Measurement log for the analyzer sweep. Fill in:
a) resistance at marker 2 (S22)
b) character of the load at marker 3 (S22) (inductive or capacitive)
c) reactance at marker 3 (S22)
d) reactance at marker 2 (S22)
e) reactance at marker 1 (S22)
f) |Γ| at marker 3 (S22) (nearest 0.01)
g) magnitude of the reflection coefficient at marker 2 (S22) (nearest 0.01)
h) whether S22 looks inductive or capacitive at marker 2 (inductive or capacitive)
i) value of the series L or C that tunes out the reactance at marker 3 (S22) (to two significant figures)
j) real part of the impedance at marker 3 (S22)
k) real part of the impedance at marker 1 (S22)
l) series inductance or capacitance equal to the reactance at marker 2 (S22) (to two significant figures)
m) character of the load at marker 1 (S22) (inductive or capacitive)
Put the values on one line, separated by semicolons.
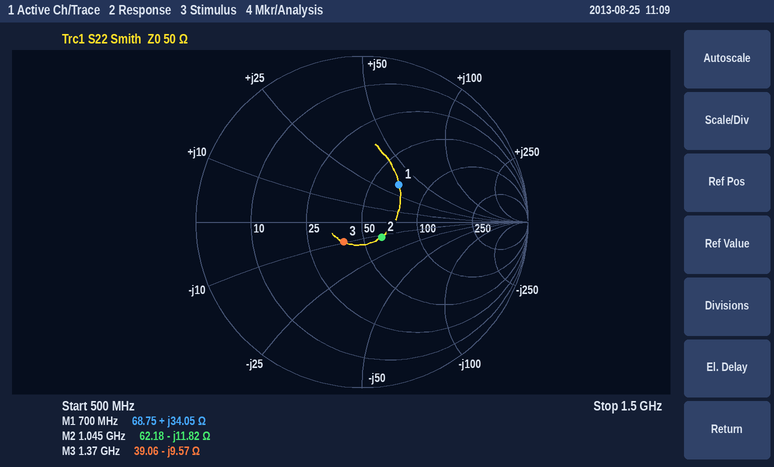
62.18 Ω; capacitive; -9.57 Ω; -11.82 Ω; +34.05 Ω; 0.16; 0.15; capacitive; 1.1 nH; 39.06 Ω; 68.75 Ω; 13 pF; inductive
